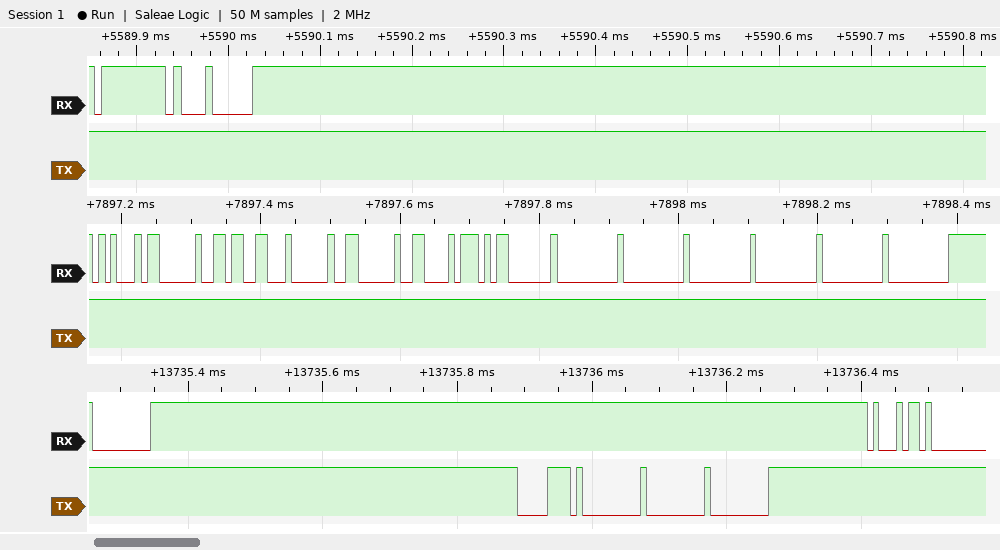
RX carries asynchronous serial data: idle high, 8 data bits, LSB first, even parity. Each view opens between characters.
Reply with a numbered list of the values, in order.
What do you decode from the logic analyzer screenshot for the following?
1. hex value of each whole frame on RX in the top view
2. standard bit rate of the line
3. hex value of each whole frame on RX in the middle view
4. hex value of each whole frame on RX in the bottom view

1. FF, 04
2. 115200 baud
3. 45, 20, 33, 20, 20, E8, 03, 00, 00, 00, 00, 00, 00
4. 00, D1
